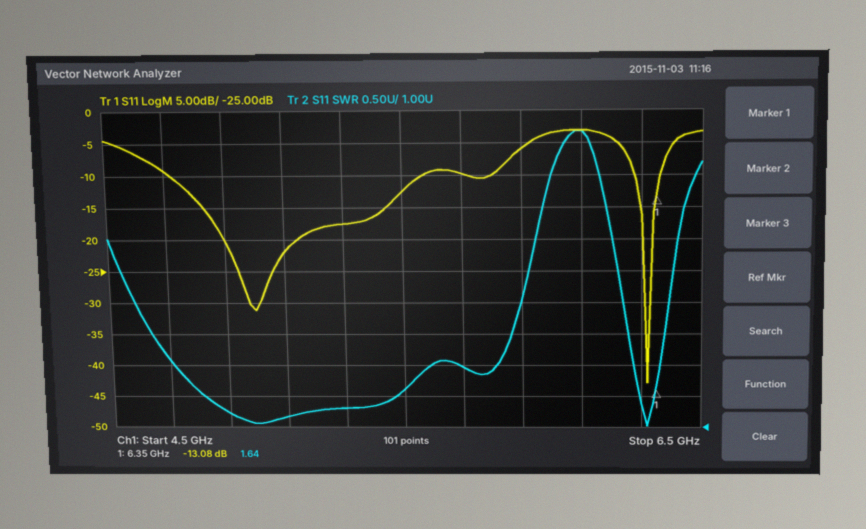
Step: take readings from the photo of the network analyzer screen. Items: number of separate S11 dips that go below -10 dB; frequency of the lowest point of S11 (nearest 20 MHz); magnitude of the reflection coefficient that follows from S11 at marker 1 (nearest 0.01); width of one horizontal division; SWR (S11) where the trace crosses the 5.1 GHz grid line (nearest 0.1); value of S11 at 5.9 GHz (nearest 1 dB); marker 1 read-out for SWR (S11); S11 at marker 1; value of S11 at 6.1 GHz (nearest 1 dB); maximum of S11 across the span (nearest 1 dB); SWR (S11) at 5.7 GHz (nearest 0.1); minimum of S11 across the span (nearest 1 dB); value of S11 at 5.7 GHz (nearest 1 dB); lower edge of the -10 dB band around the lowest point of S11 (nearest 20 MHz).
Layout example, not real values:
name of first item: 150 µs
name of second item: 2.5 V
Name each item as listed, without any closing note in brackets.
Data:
number of separate S11 dips that go below -10 dB: 2
frequency of the lowest point of S11: 6.32 GHz
magnitude of the reflection coefficient that follows from S11 at marker 1: 0.22
width of one horizontal division: 200 MHz
SWR (S11) where the trace crosses the 5.1 GHz grid line: 1.2
value of S11 at 5.9 GHz: -6 dB
marker 1 read-out for SWR: 1.64
S11 at marker 1: -13.08 dB
value of S11 at 6.1 GHz: -3 dB
maximum of S11 across the span: -3 dB
SWR (S11) at 5.7 GHz: 2.0
minimum of S11 across the span: -43 dB
value of S11 at 5.7 GHz: -10 dB
lower edge of the -10 dB band around the lowest point of S11: 6.28 GHz
